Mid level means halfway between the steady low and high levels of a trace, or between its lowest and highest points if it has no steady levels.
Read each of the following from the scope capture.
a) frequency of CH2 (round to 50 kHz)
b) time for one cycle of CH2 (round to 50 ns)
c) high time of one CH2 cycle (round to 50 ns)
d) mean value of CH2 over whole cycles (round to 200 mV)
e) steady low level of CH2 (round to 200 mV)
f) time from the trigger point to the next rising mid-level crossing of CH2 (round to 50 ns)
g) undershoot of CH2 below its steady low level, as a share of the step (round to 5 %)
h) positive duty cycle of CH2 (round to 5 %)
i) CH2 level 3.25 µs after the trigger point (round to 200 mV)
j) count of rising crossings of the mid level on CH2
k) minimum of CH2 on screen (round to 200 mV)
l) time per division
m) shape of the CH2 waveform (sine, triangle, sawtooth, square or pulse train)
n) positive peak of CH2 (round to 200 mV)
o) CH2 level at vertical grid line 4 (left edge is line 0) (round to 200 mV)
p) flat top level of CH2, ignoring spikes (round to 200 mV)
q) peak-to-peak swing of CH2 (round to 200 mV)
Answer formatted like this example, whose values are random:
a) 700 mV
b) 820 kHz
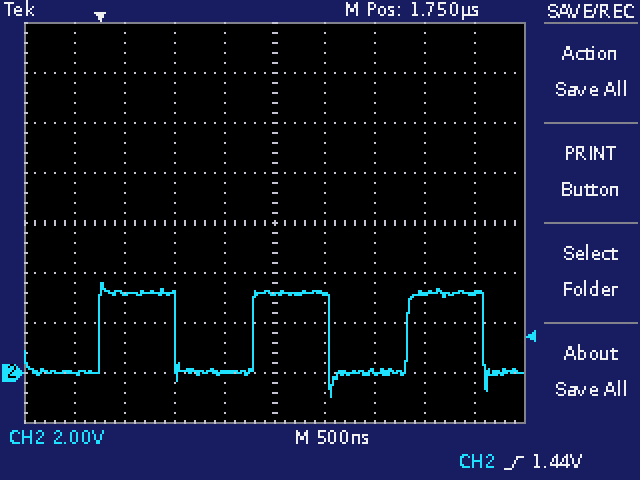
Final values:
a) 650 kHz
b) 1.55 µs
c) 750 ns
d) 1.6 V
e) 0.0 V
f) 1.55 µs
g) 30 %
h) 50 %
i) 3.2 V
j) 3
k) -1.0 V
l) 500 ns
m) square
n) 3.6 V
o) 0.0 V
p) 3.2 V
q) 4.6 V
